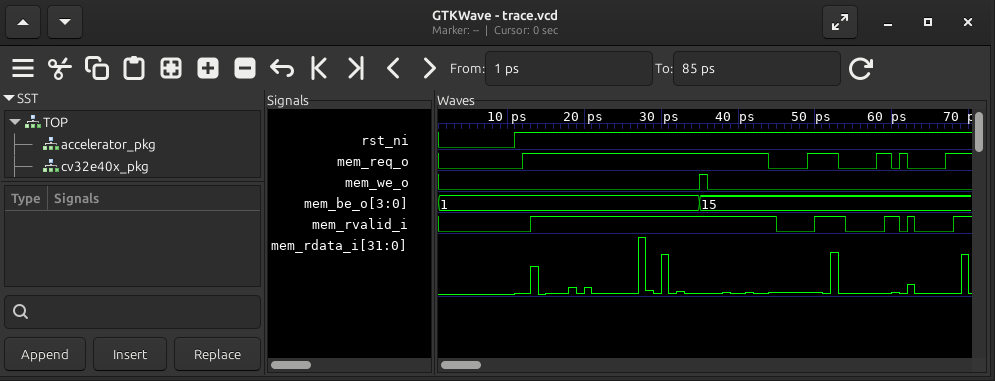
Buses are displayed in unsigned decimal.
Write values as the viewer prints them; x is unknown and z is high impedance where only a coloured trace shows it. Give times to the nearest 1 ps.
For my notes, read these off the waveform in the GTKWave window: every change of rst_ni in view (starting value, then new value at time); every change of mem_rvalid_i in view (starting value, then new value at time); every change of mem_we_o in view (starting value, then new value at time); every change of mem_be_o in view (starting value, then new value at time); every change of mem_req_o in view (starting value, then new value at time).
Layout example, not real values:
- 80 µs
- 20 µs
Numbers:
- 0, 1 at 11 ps
- 0, 1 at 13 ps, 0 at 45 ps, 1 at 50 ps, 0 at 54 ps, 1 at 59 ps, 0 at 61 ps, 1 at 62 ps, 0 at 63 ps, 1 at 68 ps
- 0, 1 at 35 ps, 0 at 36 ps
- 1, 15 at 35 ps
- 0, 1 at 12 ps, 0 at 44 ps, 1 at 49 ps, 0 at 53 ps, 1 at 58 ps, 0 at 60 ps, 1 at 61 ps, 0 at 62 ps, 1 at 67 ps
